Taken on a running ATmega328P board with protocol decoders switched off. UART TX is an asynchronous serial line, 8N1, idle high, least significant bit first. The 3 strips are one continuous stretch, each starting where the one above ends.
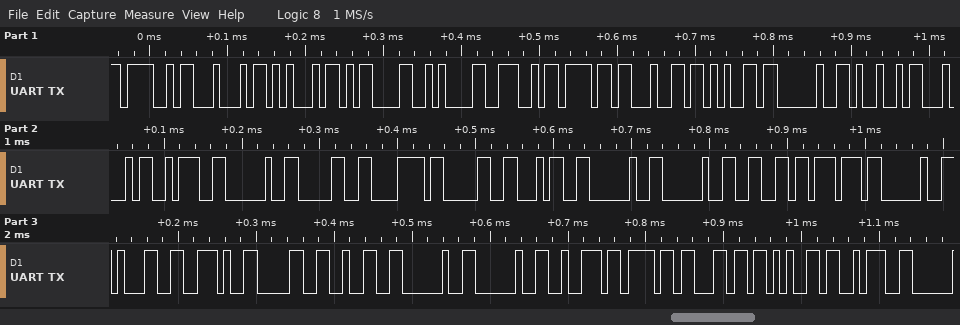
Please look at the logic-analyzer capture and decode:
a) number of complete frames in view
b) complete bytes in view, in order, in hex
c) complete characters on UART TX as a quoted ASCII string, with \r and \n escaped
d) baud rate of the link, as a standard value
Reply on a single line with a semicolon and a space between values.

34; 0x4F 0x44 0x45 0x0D 0x0A 0x4E 0x6F 0x64 0x65 0x20 0x49 0x44 0x3A 0x20 0x30 0x78 0x30 0x34 0x20 0x20 0x66 0x77 0x20 0x31 0x2E 0x30 0x32 0x20 0x20 0x72 0x6F 0x6C 0x65 0x3A; "ODE\r\nNode ID: 0x04  fw 1.02  role:"; 115200 baud
